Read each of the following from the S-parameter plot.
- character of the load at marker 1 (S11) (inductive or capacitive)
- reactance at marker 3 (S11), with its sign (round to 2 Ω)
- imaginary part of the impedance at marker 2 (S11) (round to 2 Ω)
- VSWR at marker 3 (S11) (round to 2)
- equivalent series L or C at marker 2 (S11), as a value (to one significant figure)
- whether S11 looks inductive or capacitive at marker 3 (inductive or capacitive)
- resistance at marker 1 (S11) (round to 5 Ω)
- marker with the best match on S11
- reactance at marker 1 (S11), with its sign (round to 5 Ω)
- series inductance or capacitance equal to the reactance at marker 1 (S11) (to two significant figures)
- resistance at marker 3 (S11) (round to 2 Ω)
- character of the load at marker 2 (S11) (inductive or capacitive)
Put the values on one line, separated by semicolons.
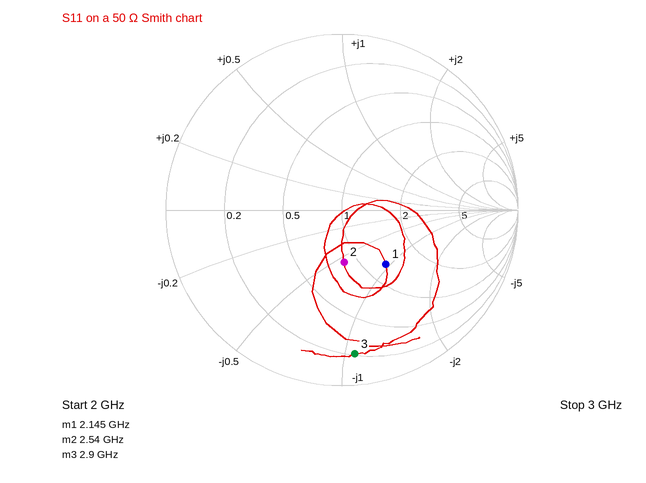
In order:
capacitive; -54 Ω; -28 Ω; 10; 2 pF; capacitive; 65 Ω; marker 2; -45 Ω; 1.6 pF; 10 Ω; capacitive
